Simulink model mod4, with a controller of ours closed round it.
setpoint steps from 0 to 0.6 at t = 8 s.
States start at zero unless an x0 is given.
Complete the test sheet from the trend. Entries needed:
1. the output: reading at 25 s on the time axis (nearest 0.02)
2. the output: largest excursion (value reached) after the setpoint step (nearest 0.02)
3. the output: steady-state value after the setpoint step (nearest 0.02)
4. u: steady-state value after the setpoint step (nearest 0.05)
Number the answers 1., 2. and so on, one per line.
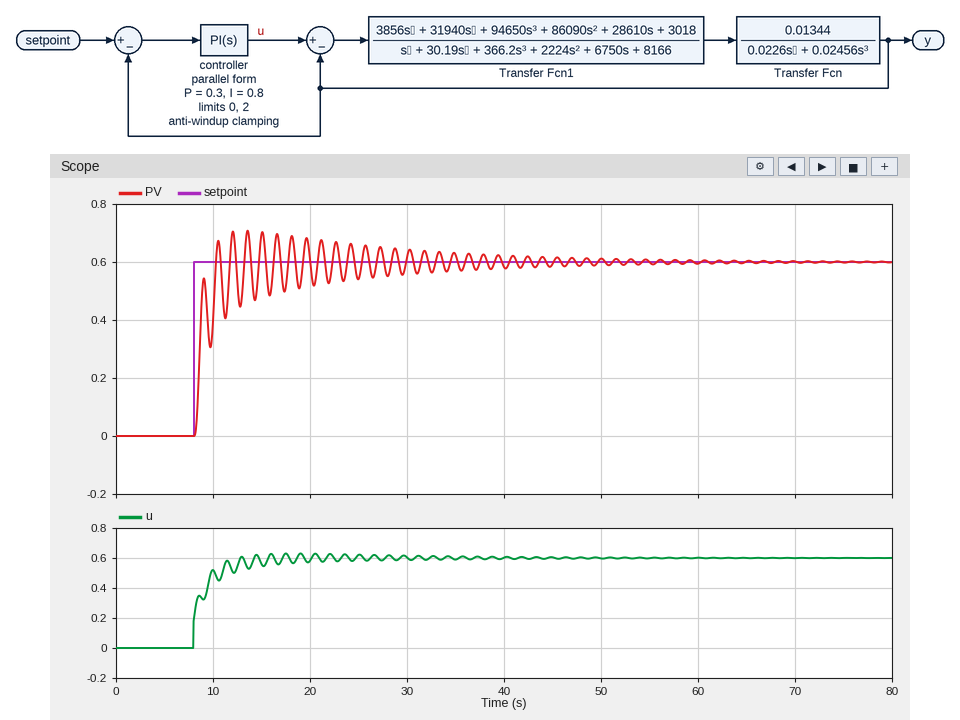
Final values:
1. 0.54
2. 0.70
3. 0.60
4. 0.60
